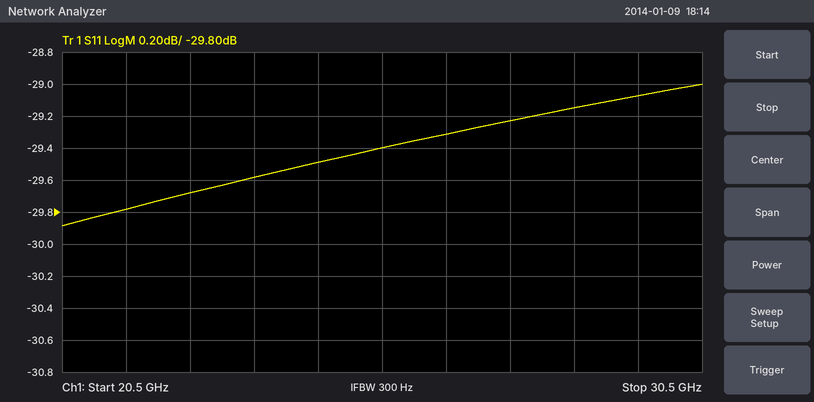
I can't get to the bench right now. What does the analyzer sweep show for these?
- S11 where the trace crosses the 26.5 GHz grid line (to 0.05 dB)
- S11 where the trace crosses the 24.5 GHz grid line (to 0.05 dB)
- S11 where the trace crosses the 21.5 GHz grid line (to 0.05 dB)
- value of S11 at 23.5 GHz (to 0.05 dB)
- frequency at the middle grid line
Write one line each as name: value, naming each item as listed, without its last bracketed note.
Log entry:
S11 where the trace crosses the 26.5 GHz grid line: -29.30 dB
S11 where the trace crosses the 24.5 GHz grid line: -29.50 dB
S11 where the trace crosses the 21.5 GHz grid line: -29.80 dB
value of S11 at 23.5 GHz: -29.60 dB
frequency at the middle grid line: 25.5 GHz
